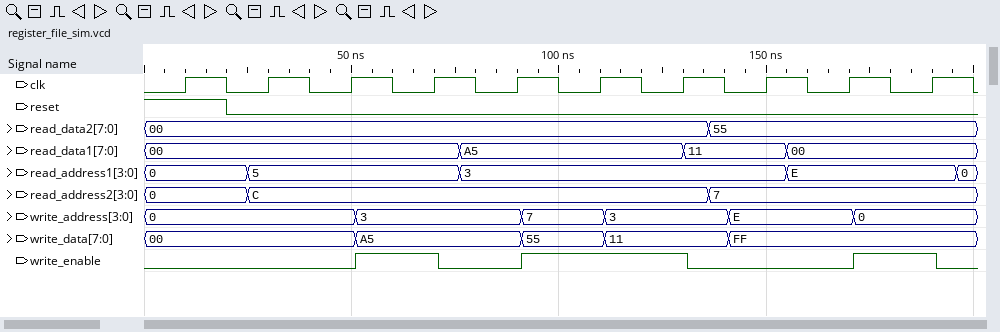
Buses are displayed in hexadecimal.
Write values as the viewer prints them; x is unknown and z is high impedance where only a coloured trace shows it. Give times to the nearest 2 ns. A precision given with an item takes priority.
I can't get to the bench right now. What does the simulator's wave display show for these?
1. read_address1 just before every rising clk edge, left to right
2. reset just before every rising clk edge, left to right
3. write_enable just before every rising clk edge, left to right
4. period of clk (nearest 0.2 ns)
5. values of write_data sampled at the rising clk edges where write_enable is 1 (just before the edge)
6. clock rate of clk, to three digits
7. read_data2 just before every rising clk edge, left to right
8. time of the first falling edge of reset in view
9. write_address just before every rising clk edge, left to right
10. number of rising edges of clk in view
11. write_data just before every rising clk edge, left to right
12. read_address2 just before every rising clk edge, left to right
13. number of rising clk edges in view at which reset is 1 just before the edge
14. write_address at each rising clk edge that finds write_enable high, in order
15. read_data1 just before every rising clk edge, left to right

0, 5, 5, 5, 3, 3, 3, 3, E, E
1 0 0 0 0 0 0 0 0 0
0 0 0 1 0 1 1 0 0 1
20 ns
A5, 55, 11, FF
50.0 MHz
00, 00, 00, 00, 00, 00, 00, 55, 55, 55
20 ns
0, 0, 0, 3, 3, 7, 3, E, E, 0
10
00, 00, 00, A5, A5, 55, 11, FF, FF, FF
0, C, C, C, C, C, C, 7, 7, 7
1
3, 7, 3, 0
00, 00, 00, 00, A5, A5, A5, 11, 00, 00
